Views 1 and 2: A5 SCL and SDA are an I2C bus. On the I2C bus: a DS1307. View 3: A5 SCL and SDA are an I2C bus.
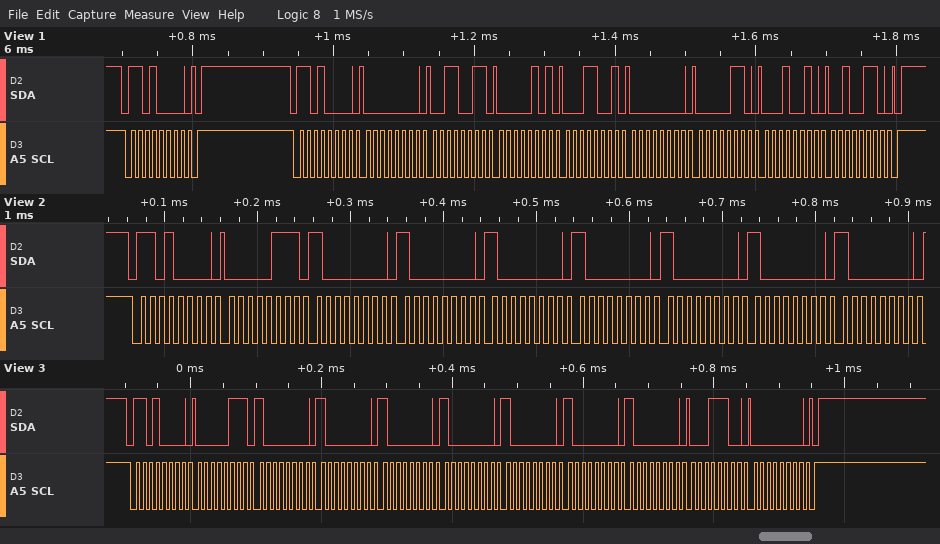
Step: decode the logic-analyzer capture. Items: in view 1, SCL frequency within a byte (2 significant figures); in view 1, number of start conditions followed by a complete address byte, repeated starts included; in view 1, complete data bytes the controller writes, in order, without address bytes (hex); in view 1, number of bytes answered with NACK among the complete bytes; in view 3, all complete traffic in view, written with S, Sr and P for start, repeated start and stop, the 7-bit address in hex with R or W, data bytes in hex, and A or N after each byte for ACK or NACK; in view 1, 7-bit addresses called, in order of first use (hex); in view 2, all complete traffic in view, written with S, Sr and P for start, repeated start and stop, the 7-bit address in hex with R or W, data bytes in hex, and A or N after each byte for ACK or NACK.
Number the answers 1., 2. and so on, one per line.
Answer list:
1. 100 kHz
2. 2
3. 00 33 05 19 00 06 12 26
4. 0
5. S 68W A 07 A 80 A 80 A 80 A 80 A 80 A 80 A 80 A 1C A 00 A P
6. 0x68
7. S 68W A 07 A 80 A 80 A 80 A 80 A 80 A 80 A 80 A
